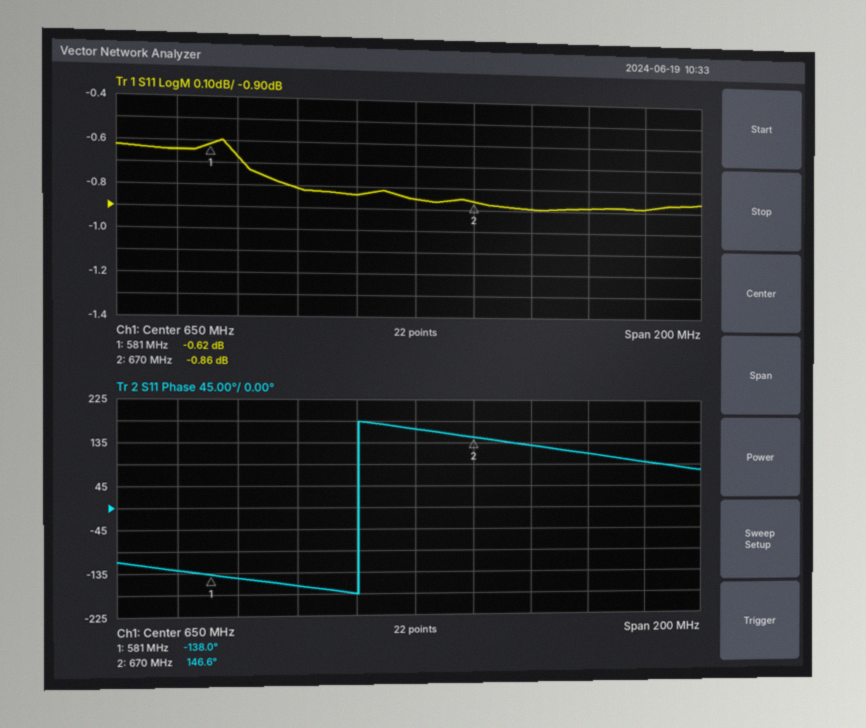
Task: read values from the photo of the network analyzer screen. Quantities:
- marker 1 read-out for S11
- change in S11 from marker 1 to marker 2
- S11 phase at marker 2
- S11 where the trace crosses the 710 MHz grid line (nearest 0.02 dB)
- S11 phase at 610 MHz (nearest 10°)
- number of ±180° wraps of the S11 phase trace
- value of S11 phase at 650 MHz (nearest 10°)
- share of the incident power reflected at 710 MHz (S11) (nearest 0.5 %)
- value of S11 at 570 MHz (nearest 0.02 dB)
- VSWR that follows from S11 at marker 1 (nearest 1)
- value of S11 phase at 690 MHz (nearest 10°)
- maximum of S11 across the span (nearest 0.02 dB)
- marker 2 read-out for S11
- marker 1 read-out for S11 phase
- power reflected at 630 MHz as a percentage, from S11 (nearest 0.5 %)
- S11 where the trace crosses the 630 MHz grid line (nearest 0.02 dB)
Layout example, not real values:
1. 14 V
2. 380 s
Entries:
1. -0.62 dB
2. -0.24 dB
3. 146.6°
4. -0.88 dB
5. -160°
6. 1
7. 160°
8. 81.5 %
9. -0.64 dB
10. 28
11. 130°
12. -0.60 dB
13. -0.86 dB
14. -138.0°
15. 82.5 %
16. -0.84 dB
